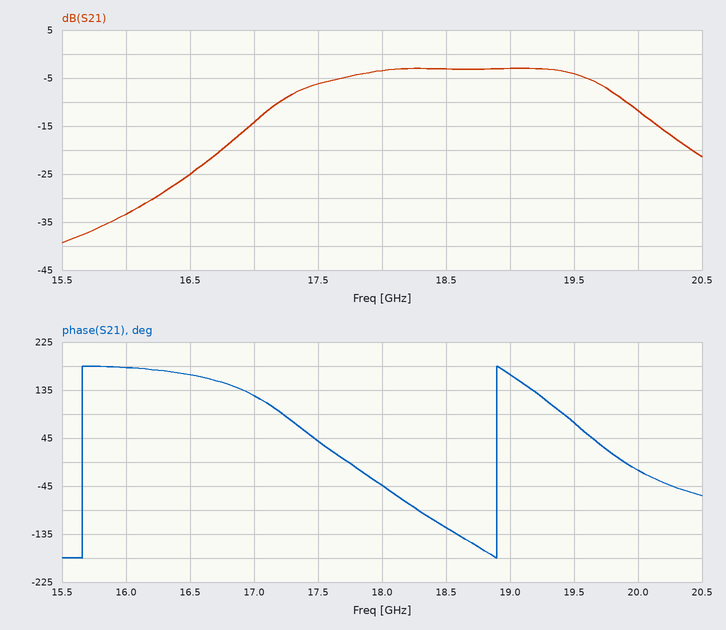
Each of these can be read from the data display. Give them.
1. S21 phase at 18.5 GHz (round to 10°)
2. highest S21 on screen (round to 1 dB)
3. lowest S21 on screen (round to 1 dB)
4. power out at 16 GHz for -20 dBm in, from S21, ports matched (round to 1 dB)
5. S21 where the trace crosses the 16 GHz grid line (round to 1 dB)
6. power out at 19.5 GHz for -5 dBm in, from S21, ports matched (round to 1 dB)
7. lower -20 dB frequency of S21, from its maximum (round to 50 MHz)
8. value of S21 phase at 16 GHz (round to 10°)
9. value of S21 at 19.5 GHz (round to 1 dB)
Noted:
-120°
-3 dB
-39 dB
-53 dBm
-33 dB
-9 dBm
16.60 GHz
180°
-4 dB
